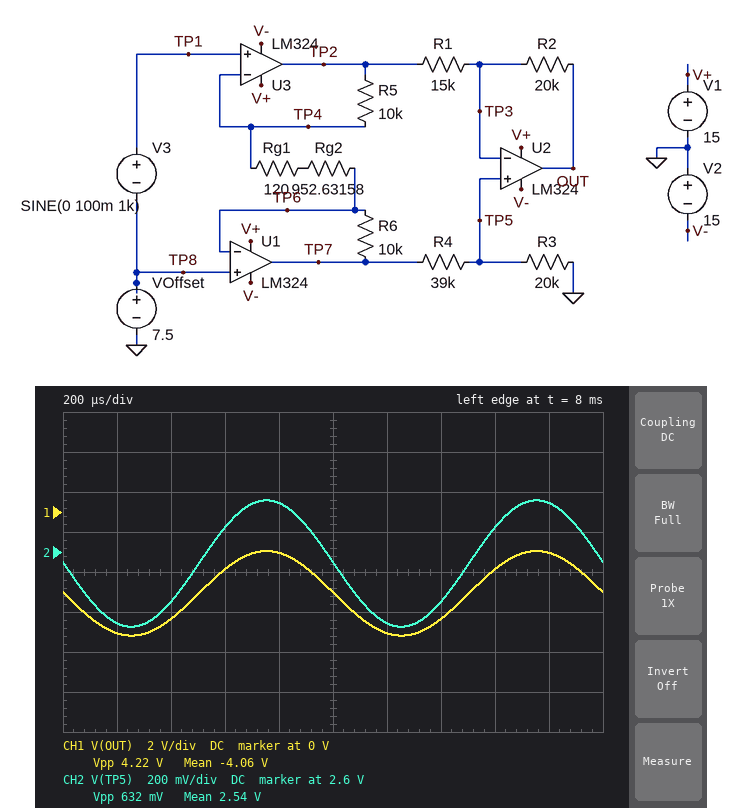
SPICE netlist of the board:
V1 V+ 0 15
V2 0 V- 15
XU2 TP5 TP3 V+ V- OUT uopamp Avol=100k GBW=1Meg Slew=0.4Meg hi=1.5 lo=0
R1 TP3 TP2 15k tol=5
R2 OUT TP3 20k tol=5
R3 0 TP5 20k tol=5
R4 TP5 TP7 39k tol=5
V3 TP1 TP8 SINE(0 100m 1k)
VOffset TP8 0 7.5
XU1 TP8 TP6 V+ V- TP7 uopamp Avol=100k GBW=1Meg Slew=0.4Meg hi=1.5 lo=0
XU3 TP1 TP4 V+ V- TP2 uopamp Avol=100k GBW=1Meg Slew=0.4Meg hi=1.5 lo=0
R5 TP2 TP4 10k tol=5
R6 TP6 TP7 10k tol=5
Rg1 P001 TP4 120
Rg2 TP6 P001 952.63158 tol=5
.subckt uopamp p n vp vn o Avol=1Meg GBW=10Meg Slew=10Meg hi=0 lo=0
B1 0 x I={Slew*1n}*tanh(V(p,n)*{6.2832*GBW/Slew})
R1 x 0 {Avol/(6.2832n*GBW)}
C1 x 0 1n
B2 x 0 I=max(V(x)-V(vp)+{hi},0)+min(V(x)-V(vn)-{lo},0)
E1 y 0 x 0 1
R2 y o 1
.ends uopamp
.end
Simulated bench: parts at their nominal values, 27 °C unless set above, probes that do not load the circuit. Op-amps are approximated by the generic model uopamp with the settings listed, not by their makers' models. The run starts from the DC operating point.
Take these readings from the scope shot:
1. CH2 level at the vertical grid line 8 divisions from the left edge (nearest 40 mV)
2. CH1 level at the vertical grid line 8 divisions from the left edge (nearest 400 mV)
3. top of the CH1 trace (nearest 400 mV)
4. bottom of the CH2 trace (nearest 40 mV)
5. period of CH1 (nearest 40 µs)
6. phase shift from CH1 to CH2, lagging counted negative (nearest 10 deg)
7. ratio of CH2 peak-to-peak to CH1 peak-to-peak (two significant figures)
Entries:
2.72 V
-2.8 V
-2.0 V
2.24 V
1.00 ms
0 deg
0.15
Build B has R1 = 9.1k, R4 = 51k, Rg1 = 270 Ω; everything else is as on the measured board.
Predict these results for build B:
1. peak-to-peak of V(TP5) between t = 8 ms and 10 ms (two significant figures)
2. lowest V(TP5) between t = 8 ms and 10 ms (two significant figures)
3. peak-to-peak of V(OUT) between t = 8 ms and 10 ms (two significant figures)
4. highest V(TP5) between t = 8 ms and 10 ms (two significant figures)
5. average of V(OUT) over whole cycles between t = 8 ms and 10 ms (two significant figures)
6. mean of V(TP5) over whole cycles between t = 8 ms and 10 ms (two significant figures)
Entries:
460 mV
1.9 V
5.5 V
2.3 V
-9.7 V
2.1 V
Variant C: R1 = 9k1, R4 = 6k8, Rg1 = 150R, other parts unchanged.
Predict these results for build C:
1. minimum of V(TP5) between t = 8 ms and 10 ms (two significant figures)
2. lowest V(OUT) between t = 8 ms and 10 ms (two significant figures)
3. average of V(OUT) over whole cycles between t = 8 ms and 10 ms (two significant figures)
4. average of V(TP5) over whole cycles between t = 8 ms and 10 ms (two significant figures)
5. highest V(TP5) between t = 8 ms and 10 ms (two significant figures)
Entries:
4.9 V
-3.0 V
1.4 V
5.6 V
6.3 V
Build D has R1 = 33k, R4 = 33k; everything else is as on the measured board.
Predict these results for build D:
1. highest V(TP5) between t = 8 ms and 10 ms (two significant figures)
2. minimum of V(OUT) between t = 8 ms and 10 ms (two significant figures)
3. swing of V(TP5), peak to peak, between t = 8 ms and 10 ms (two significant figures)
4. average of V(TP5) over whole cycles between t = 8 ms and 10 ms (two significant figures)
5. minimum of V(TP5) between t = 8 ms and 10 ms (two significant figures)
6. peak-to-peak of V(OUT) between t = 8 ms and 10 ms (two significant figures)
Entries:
3.2 V
-1.2 V
700 mV
2.8 V
2.5 V
2.4 V
